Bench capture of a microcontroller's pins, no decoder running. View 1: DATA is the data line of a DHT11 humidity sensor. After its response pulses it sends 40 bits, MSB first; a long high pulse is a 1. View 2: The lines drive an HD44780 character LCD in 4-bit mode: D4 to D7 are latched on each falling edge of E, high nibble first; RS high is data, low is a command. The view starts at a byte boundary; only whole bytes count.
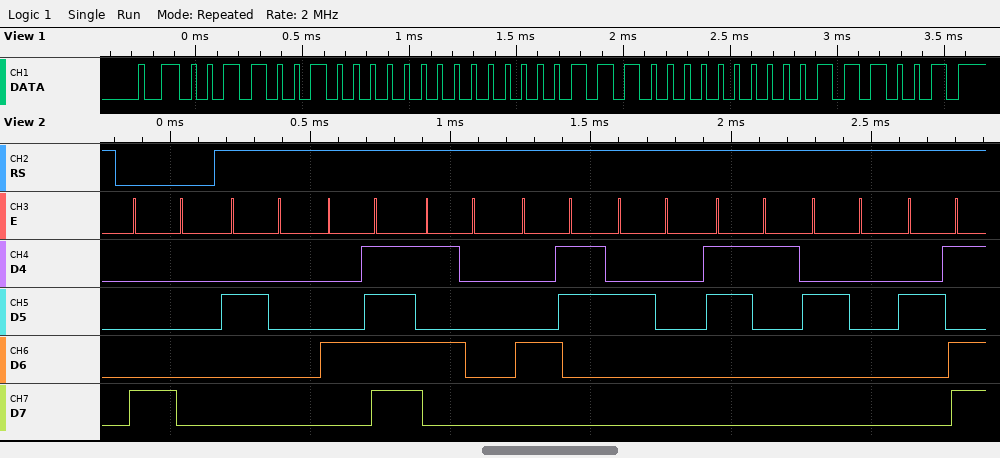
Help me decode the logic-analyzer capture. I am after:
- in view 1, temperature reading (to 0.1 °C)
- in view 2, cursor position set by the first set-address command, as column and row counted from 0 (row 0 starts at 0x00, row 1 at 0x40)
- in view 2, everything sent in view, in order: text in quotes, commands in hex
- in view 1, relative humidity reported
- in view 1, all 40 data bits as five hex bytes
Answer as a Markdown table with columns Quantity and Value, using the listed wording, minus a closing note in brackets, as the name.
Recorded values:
| Quantity | Value |
|---|---|
| in view 1, temperature reading | 7.0 °C |
| in view 2, cursor position set by the first set-address command, as column and row counted from 0 | column 0, row 0 |
| in view 2, everything sent in view, in order: text in quotes, commands in hex | 0x80 " OPC 1 -" |
| in view 1, relative humidity reported | 50 % |
| in view 1, all 40 data bits as five hex bytes | 32 00 07 00 39 |
